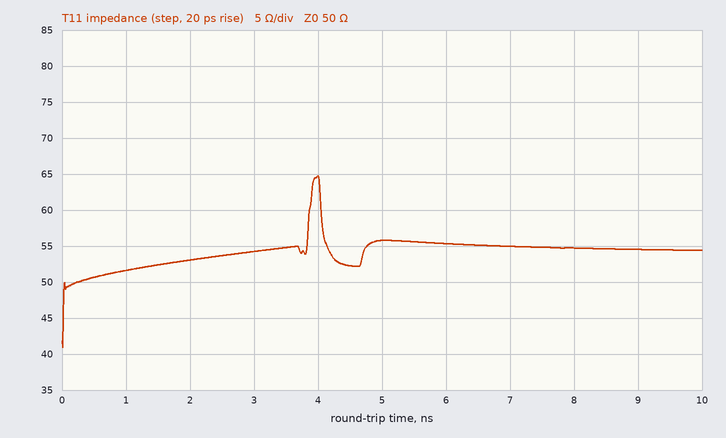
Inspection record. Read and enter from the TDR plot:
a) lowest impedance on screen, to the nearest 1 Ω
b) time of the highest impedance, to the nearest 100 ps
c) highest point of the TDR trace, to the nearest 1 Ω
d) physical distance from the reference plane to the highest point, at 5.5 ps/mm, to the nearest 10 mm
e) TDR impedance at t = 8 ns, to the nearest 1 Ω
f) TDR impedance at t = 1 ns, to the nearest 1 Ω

41 Ω
4.0 ns
65 Ω
360 mm
55 Ω
52 Ω
